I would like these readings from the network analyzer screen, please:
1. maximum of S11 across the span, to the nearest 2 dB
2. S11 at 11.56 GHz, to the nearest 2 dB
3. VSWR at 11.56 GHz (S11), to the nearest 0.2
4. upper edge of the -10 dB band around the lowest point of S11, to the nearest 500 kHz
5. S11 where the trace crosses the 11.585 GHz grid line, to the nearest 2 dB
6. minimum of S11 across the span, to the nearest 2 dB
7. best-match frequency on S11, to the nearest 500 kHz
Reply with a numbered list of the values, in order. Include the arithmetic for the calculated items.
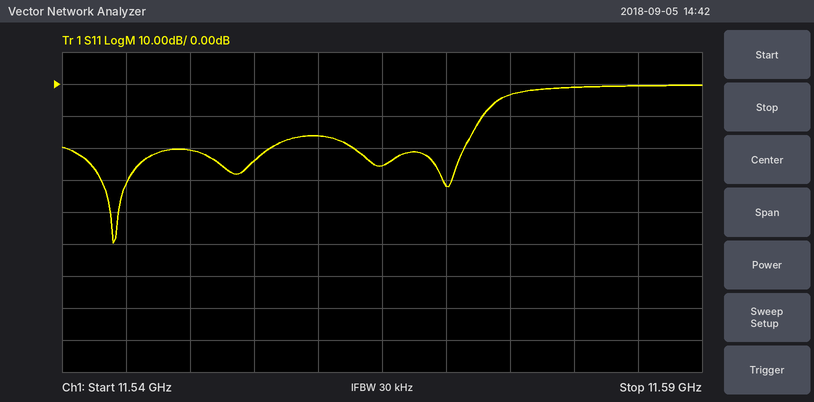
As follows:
1. 0 dB
2. -16 dB
3. |Γ| = 10^(-16/20) = 0.1585; VSWR = (1 + 0.1585)/(1 − 0.1585) ≈ 1.4
4. 11.5730 GHz
5. 0 dB
6. -50 dB
7. 11.5440 GHz
